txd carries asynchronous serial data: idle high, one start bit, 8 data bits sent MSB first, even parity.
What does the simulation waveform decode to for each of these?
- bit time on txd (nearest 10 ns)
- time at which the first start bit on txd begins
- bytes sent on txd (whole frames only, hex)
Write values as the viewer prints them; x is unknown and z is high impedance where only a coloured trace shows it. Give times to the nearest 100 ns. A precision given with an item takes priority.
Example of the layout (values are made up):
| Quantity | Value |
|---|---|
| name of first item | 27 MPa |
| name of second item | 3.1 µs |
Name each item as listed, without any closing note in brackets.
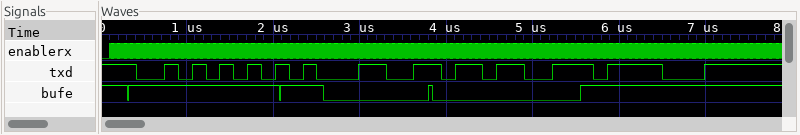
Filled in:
| Quantity | Value |
|---|---|
| bit time on txd | 160 ns |
| time at which the first start bit on txd begins | 400 ns |
| bytes sent on txd | 55, 8C, D9, F1 |
